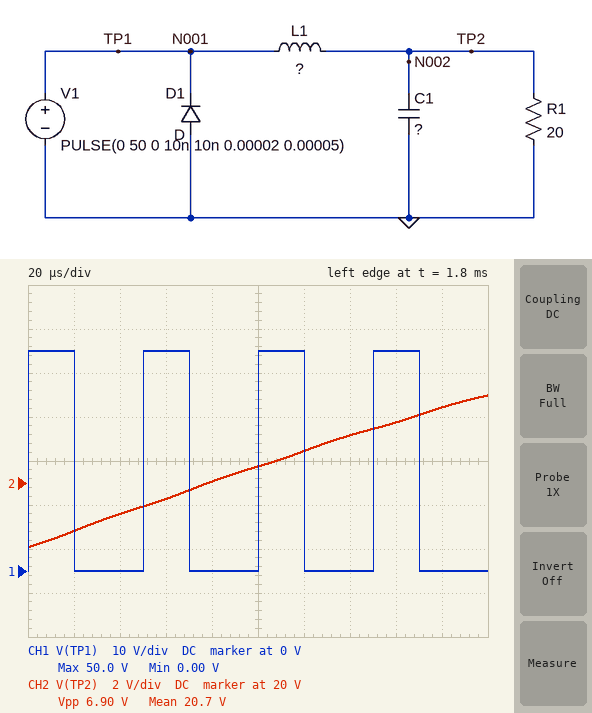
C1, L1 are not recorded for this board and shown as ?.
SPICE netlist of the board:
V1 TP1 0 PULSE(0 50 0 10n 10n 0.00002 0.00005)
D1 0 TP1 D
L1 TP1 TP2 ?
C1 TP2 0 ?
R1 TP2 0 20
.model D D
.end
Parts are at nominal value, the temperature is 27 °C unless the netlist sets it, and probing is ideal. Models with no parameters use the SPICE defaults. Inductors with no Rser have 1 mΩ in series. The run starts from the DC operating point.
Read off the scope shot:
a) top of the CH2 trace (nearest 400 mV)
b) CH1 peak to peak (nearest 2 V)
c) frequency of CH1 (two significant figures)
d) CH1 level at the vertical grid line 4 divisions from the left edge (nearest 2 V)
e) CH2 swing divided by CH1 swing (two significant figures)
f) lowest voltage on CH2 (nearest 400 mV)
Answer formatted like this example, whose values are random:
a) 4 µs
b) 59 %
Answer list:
a) 24.0 V
b) 50 V
c) 20 kHz
d) 0 V
e) 0.14
f) 17.2 V
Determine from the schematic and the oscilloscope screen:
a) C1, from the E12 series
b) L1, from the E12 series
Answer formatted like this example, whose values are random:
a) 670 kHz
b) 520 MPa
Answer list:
a) 56 µF
b) 1 mH
